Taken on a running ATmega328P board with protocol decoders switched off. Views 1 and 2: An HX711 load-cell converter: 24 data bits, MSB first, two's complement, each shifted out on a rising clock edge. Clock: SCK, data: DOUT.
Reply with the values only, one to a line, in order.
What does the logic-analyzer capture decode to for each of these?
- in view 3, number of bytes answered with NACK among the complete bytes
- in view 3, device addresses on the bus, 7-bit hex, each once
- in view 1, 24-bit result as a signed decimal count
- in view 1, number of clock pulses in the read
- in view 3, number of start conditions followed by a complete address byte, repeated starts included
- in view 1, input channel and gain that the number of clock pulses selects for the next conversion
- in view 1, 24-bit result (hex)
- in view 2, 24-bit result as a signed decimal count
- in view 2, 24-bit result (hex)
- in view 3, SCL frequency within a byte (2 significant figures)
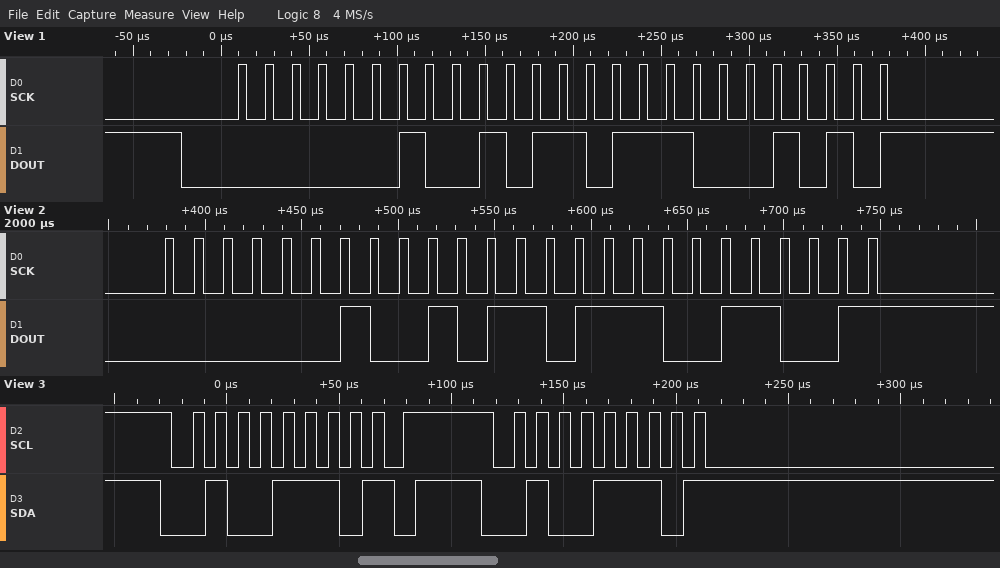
2
0x27
154506
25
2
channel A, gain 128
0x025B8A
154521
0x025B99
100 kHz
